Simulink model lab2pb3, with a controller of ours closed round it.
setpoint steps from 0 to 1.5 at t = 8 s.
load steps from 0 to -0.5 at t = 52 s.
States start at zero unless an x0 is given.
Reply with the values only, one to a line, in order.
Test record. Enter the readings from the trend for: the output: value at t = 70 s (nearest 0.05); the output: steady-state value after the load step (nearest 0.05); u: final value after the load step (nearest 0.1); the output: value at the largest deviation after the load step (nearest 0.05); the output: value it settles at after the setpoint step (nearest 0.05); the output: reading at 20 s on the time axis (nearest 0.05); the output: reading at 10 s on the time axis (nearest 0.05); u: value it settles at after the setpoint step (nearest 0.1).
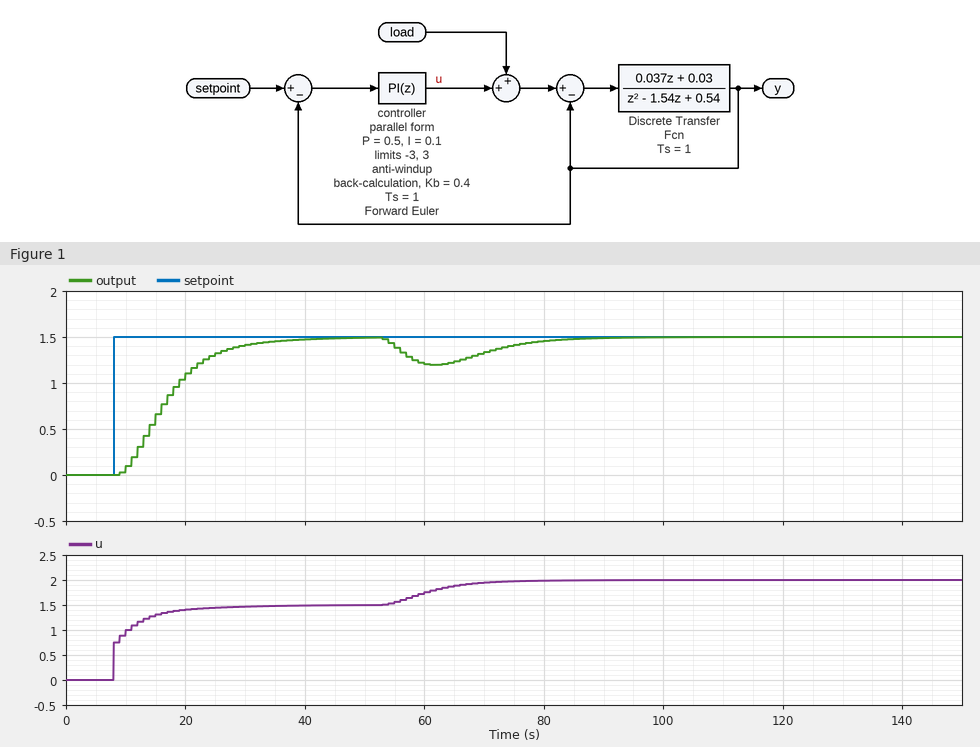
1.35
1.50
2.0
1.20
1.50
1.10
0.10
1.5
